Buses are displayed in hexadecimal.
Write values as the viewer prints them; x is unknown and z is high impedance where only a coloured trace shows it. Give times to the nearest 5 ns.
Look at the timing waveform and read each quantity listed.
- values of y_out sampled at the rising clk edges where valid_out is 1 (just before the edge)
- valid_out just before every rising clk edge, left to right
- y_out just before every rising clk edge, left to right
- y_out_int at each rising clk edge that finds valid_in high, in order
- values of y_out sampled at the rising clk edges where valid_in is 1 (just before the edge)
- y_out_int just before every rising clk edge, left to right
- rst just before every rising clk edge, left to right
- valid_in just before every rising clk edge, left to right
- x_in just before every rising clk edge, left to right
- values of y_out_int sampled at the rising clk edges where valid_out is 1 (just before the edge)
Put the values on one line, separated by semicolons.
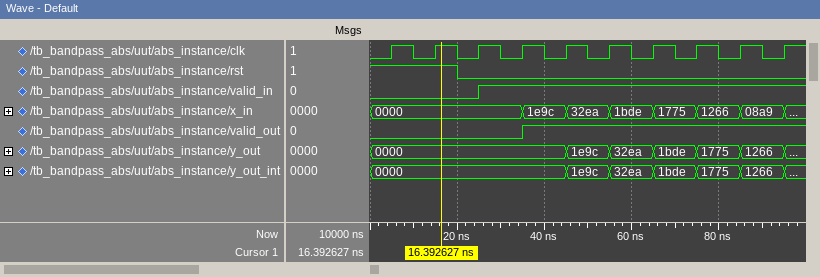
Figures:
0000, 1e9c, 32ea, 1bde, 1775, 1266; 0 0 0 0 1 1 1 1 1 1; 0000, 0000, 0000, 0000, 0000, 1e9c, 32ea, 1bde, 1775, 1266; 0000, 0000, 1e9c, 32ea, 1bde, 1775, 1266; 0000, 0000, 1e9c, 32ea, 1bde, 1775, 1266; 0000, 0000, 0000, 0000, 0000, 1e9c, 32ea, 1bde, 1775, 1266; 1 1 0 0 0 0 0 0 0 0; 0 0 0 1 1 1 1 1 1 1; 0000, 0000, 0000, 0000, 1e9c, 32ea, 1bde, 1775, 1266, 08a9; 0000, 1e9c, 32ea, 1bde, 1775, 1266
